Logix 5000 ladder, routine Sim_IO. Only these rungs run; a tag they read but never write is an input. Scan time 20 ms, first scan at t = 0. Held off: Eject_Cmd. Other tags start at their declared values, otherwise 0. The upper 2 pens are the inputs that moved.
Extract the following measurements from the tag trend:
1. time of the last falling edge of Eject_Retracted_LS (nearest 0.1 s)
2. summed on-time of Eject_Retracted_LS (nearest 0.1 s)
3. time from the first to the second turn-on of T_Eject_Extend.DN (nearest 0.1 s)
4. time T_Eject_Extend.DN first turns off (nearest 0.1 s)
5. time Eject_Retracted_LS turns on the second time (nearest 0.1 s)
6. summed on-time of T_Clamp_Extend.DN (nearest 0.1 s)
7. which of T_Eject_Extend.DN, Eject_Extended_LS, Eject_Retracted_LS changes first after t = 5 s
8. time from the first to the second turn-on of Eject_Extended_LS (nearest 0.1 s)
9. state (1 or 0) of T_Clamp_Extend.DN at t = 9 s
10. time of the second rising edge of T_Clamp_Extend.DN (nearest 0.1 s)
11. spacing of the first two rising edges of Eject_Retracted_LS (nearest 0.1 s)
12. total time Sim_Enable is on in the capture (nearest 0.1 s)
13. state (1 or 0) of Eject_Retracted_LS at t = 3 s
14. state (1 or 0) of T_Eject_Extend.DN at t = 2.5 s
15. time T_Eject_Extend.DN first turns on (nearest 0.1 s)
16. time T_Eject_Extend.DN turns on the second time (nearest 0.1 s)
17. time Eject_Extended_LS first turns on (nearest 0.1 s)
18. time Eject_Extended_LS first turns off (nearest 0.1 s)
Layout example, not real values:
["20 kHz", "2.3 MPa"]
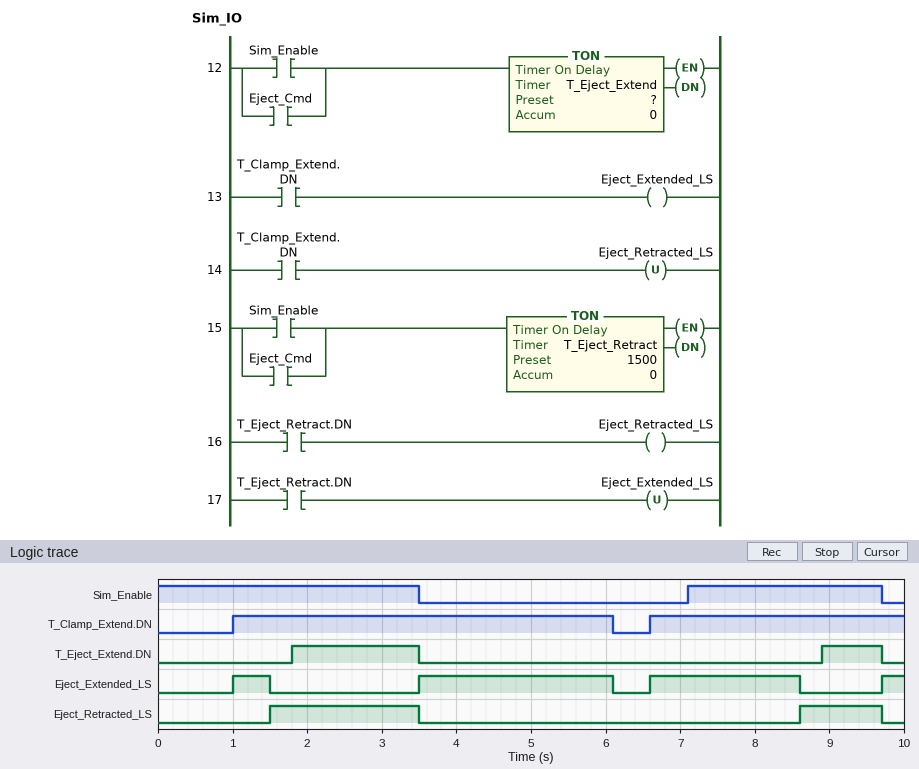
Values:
["9.7 s", "3.1 s", "7.1 s", "3.5 s", "8.6 s", "8.5 s", "Eject_Extended_LS", "2.5 s", "1", "6.6 s", "7.1 s", "6.1 s", "1", "1", "1.8 s", "8.9 s", "1.0 s", "1.5 s"]
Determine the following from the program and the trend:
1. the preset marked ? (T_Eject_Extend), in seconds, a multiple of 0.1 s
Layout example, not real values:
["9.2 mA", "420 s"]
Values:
["1.8 s"]
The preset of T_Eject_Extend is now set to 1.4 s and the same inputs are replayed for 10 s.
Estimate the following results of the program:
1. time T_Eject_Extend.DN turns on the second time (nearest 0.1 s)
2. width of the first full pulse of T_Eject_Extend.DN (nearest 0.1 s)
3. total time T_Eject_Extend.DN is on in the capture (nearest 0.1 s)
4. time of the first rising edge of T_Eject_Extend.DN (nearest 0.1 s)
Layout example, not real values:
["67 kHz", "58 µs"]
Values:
["8.5 s", "2.1 s", "3.3 s", "1.4 s"]
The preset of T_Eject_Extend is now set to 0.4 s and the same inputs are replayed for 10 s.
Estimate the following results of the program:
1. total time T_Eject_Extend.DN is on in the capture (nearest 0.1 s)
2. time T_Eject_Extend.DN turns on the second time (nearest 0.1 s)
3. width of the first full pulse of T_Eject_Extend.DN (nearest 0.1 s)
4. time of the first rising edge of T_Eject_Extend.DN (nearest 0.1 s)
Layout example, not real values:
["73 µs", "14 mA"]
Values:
["5.3 s", "7.5 s", "3.1 s", "0.4 s"]
